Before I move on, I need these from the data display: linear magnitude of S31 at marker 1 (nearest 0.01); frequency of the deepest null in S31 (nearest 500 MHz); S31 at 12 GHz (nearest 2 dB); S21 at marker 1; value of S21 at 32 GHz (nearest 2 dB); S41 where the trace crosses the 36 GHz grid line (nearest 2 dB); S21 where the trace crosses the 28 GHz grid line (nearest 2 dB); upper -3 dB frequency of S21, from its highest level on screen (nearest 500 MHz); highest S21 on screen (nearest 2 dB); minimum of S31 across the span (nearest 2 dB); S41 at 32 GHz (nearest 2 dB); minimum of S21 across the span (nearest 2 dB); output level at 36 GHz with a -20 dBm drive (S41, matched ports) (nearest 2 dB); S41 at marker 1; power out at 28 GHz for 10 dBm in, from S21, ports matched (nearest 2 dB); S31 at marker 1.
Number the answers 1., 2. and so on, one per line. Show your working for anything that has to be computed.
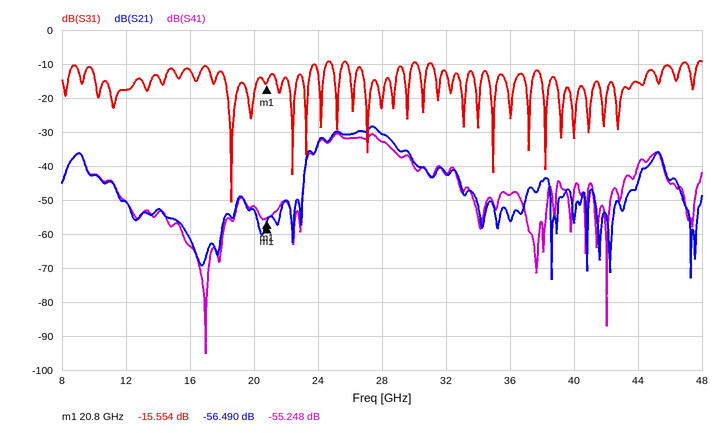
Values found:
1. 10^(-15.554/20) ≈ 0.17
2. 18.5 GHz
3. -18 dB
4. -56.490 dB
5. -42 dB
6. -48 dB
7. -30 dB
8. 28.5 GHz
9. -28 dB
10. -50 dB
11. -42 dB
12. -74 dB
13. -20 dBm + (-48 dB) = -68 dBm
14. -55.248 dB
15. 10 dBm + (-30 dB) = -20 dBm
16. -15.554 dB
